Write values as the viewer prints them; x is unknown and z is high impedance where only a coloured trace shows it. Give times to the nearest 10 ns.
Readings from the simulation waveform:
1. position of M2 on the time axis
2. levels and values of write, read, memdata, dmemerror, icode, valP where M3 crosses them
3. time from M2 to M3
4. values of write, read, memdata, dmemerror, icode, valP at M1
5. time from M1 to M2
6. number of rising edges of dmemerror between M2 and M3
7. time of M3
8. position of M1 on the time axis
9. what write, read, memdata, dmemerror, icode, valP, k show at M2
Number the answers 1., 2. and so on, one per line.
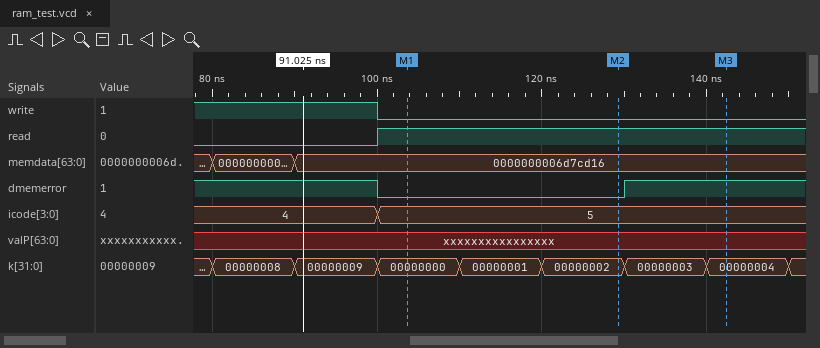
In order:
1. 130 ns
2. write=0, read=1, memdata=0000000006d7cd16, dmemerror=1, icode=5, valP=xxxxxxxxxxxxxxxx
3. 10 ns
4. write=0, read=1, memdata=0000000006d7cd16, dmemerror=0, icode=5, valP=xxxxxxxxxxxxxxxx
5. 30 ns
6. 1
7. 140 ns
8. 100 ns
9. write=0, read=1, memdata=0000000006d7cd16, dmemerror=0, icode=5, valP=xxxxxxxxxxxxxxxx, k=00000002
